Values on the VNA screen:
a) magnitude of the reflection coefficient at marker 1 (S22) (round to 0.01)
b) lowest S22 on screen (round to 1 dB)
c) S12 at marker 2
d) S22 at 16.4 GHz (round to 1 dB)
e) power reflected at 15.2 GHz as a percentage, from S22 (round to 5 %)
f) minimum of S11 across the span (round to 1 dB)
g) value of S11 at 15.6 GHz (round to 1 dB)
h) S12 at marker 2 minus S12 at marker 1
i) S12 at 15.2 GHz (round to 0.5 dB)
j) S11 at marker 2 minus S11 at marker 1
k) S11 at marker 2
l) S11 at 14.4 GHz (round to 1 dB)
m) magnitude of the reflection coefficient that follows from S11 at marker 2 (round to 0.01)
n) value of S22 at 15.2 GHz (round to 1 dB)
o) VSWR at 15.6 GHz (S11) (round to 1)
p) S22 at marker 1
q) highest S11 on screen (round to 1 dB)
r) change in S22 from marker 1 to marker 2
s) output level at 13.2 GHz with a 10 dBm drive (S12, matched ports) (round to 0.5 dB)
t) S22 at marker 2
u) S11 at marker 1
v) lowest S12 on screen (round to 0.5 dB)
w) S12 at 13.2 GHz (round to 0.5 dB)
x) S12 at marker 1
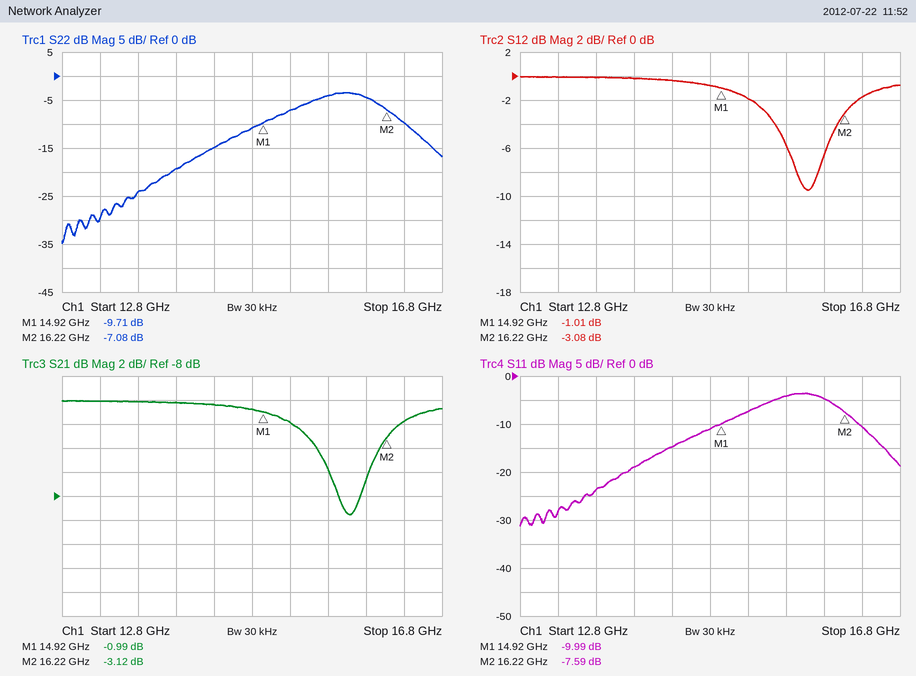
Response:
0.33
-35 dB
-3.08 dB
-10 dB
20 %
-31 dB
-4 dB
-2.07 dB
-2.0 dB
2.40 dB
-7.59 dB
-15 dB
0.42
-7 dB
4
-9.71 dB
-4 dB
2.63 dB
10.0 dBm
-7.08 dB
-9.99 dB
-9.5 dB
0.0 dB
-1.01 dB
